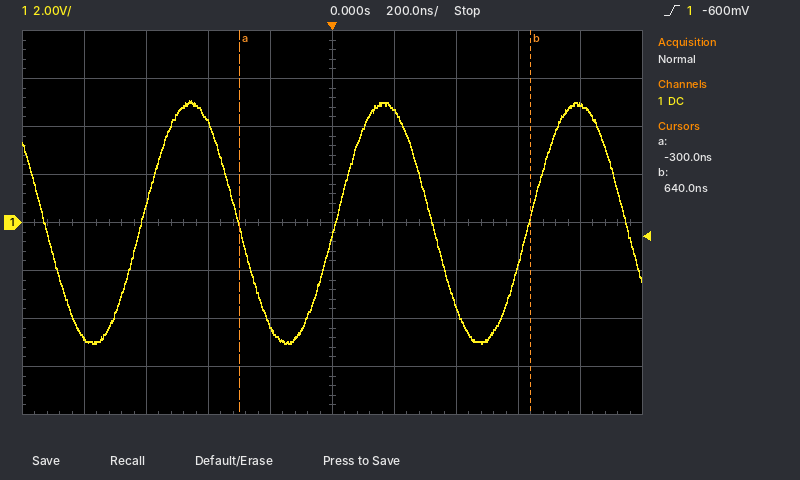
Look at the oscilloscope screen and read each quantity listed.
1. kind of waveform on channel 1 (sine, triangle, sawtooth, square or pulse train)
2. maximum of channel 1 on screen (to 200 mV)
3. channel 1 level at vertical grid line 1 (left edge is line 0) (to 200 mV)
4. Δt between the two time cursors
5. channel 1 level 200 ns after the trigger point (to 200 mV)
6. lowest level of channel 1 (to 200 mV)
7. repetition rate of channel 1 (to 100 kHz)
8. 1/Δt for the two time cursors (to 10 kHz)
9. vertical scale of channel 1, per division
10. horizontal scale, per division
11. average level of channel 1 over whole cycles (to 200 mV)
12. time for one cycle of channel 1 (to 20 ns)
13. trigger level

sine
5.0 V
-4.8 V
940 ns
4.6 V
-5.0 V
1.6 MHz
1.06 MHz
2 V
200 ns
0.0 V
620 ns
-600 mV
